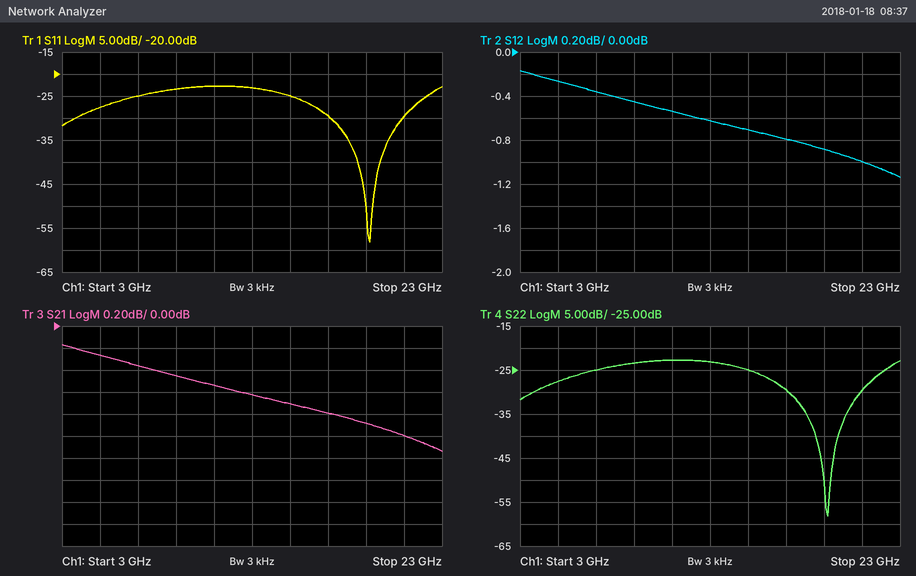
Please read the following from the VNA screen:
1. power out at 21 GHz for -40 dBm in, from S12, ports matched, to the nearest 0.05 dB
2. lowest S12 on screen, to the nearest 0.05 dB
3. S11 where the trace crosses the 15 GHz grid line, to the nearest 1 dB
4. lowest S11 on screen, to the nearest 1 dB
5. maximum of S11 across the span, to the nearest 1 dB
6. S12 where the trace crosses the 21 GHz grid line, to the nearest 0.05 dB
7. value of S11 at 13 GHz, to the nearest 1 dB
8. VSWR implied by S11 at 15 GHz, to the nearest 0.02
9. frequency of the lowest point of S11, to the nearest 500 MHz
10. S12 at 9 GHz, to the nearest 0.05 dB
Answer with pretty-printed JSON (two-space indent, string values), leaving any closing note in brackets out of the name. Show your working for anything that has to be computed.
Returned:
{
  "power out at 21 GHz for -40 dBm in, from S12, ports matched, to the nearest 0.05 dB": "-40 dBm + (-1.00 dB) = -41.00 dBm",
  "lowest S12 on screen, to the nearest 0.05 dB": "-1.15 dB",
  "S11 where the trace crosses the 15 GHz grid line, to the nearest 1 dB": "-25 dB",
  "lowest S11 on screen, to the nearest 1 dB": "-58 dB",
  "maximum of S11 across the span, to the nearest 1 dB": "-23 dB",
  "S12 where the trace crosses the 21 GHz grid line, to the nearest 0.05 dB": "-1.00 dB",
  "value of S11 at 13 GHz, to the nearest 1 dB": "-23 dB",
  "VSWR implied by S11 at 15 GHz, to the nearest 0.02": "|Γ| = 10^(-25/20) = 0.0562; VSWR = (1 + 0.0562)/(1 − 0.0562) ≈ 1.12",
  "frequency of the lowest point of S11, to the nearest 500 MHz": "19.0 GHz",
  "S12 at 9 GHz, to the nearest 0.05 dB": "-0.45 dB"
}
